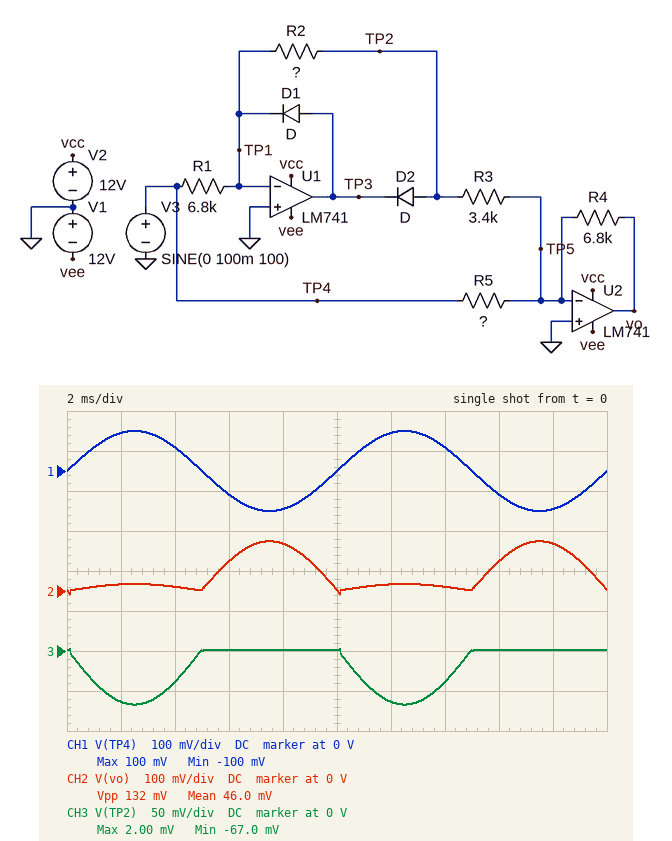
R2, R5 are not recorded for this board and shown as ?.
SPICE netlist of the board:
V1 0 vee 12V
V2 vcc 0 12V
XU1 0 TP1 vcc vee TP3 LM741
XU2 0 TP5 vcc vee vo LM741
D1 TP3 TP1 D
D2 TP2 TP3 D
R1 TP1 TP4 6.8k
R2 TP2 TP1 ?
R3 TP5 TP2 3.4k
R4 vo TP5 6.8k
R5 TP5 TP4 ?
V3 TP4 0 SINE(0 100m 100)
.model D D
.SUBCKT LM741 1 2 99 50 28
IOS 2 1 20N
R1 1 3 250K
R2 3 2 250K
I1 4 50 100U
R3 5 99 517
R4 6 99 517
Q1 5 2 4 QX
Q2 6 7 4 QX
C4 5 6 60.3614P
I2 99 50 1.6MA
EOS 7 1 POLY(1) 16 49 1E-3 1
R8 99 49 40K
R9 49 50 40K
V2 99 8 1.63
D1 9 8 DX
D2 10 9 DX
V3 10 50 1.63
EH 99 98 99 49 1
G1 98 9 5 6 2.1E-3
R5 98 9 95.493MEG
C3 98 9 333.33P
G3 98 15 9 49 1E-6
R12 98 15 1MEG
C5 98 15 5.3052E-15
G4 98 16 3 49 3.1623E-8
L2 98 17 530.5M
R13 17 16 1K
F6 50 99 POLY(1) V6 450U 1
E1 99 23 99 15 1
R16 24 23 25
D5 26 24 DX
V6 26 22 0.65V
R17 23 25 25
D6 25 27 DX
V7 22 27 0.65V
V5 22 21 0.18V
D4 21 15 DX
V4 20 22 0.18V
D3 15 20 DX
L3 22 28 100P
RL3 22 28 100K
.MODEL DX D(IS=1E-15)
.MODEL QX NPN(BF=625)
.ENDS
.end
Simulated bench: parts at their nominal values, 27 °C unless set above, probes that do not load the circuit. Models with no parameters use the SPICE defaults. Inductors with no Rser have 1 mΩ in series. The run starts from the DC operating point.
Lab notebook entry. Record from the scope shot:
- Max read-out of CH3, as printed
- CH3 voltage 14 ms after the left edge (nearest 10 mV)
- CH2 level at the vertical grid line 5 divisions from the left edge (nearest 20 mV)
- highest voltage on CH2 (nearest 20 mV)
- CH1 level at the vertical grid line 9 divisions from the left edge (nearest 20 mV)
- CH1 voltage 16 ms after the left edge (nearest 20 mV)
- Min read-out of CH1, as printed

2.00 mV
-40 mV
0 V
120 mV
-100 mV
-60 mV
-100 mV
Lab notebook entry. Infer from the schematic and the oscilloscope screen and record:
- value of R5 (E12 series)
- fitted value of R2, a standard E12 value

5.6 kΩ
4.7 kΩ
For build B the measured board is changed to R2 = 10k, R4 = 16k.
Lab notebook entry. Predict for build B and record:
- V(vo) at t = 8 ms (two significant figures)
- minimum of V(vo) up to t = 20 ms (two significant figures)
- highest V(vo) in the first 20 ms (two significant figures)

280 mV
-17 mV
400 mV
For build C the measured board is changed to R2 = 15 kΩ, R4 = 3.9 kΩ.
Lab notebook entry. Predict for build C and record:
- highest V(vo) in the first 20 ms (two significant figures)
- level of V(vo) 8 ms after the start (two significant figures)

180 mV
68 mV
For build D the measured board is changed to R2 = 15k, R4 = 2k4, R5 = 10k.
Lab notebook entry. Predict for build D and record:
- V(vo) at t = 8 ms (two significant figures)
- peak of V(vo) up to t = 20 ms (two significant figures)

24 mV
130 mV
